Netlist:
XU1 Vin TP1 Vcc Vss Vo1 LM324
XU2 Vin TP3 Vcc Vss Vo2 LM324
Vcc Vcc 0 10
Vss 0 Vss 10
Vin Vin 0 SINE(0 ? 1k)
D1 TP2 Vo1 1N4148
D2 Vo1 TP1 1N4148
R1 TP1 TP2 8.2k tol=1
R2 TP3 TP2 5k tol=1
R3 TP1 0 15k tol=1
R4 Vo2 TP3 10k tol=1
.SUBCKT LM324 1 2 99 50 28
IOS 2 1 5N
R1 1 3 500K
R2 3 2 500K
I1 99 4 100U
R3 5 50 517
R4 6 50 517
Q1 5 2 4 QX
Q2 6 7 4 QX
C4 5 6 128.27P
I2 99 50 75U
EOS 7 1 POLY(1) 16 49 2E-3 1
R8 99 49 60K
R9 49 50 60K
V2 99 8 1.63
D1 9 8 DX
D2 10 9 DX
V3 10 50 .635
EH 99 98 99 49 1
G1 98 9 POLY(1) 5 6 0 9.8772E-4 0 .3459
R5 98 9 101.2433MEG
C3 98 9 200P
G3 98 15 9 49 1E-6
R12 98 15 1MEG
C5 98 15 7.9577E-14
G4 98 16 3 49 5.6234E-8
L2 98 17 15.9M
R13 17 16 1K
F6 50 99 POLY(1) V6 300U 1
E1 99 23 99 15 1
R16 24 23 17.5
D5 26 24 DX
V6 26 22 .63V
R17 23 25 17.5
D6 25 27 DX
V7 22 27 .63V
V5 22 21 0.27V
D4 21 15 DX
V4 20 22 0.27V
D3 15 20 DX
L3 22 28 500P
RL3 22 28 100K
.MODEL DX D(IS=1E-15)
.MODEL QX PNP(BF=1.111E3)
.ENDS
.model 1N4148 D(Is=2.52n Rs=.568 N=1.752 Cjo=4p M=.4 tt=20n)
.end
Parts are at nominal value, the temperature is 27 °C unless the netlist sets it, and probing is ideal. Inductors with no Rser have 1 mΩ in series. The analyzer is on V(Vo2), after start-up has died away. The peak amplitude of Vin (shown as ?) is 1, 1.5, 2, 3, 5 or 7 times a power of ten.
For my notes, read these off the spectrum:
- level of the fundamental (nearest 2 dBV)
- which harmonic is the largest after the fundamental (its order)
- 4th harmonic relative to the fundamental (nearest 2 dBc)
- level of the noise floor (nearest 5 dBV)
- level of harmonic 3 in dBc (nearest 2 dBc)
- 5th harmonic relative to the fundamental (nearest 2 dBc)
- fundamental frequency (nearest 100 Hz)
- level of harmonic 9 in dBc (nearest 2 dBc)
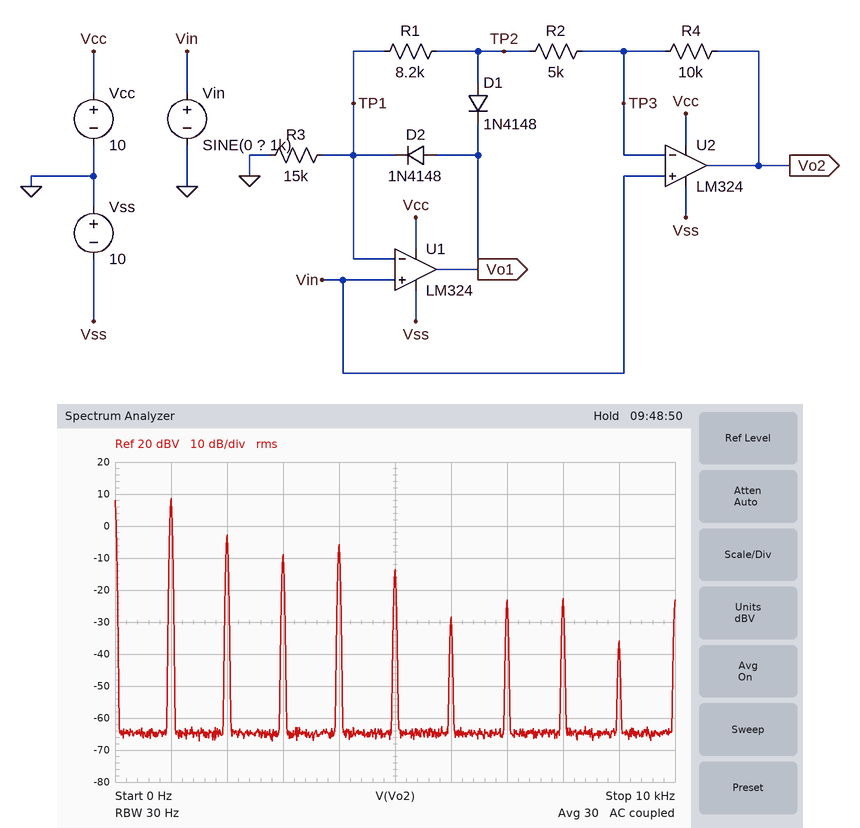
8 dBV
2
-14 dBc
-65 dBV
-18 dBc
-22 dBc
1.0 kHz
-44 dBc
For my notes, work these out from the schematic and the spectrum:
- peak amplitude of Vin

7 V
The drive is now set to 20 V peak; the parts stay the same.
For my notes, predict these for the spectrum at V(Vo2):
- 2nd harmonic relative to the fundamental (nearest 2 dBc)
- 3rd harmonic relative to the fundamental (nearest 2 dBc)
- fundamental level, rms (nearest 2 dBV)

14 dBc
8 dBc
-4 dBV
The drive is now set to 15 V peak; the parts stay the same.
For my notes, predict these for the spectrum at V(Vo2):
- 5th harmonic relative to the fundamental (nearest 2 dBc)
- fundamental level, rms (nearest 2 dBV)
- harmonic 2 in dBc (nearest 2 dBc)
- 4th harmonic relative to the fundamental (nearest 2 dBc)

-6 dBc
2 dBV
8 dBc
-20 dBc
